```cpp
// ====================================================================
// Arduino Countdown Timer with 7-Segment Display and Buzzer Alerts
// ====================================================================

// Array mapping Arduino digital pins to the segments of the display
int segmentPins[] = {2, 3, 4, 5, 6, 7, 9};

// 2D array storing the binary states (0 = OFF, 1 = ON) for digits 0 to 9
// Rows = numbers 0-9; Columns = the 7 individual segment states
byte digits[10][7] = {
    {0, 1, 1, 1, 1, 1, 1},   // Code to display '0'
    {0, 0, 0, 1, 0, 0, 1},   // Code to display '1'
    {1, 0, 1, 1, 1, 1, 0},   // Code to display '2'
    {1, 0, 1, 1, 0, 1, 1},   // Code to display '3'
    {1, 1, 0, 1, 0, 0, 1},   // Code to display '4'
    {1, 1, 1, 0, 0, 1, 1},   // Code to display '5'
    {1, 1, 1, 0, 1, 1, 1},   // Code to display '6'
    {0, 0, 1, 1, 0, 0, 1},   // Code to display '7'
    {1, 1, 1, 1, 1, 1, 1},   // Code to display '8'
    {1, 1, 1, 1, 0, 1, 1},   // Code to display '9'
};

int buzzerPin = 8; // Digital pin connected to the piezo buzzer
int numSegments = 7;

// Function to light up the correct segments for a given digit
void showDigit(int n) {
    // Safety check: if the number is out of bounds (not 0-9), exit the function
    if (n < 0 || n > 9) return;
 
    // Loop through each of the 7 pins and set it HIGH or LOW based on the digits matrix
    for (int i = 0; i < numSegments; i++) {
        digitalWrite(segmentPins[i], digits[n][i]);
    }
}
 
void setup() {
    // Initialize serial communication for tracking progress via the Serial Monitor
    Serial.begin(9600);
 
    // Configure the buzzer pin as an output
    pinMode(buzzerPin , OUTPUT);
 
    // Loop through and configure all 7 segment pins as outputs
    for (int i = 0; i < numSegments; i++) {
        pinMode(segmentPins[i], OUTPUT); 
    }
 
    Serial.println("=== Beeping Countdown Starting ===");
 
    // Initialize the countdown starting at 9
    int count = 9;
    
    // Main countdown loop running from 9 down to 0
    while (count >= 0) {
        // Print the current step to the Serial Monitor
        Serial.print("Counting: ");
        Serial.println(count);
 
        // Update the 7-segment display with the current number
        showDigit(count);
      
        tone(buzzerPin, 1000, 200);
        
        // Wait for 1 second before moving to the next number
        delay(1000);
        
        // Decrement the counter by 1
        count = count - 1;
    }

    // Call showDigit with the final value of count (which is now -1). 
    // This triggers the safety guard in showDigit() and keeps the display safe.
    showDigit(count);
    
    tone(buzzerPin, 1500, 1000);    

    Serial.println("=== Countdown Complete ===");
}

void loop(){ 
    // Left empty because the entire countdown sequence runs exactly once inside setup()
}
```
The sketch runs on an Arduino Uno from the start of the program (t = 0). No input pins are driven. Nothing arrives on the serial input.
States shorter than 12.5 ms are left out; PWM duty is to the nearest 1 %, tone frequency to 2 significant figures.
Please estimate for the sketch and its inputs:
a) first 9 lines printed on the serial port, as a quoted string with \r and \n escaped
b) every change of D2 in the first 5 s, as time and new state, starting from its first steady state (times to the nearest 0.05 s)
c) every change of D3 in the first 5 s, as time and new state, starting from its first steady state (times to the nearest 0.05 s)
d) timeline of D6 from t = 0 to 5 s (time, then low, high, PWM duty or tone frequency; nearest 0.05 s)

"=== Beeping Countdown Starting ===\r\nCounting: 9\r\nCounting: 8\r\nCounting: 7\r\nCounting: 6\r\nCounting: 5\r\nCounting: 4\r\nCounting: 3\r\nCounting: 2\r\n"
0 s high; 2 s low; 3 s high
0 s high; 2 s low; 3 s high
0 s low; 1 s high; 2 s low; 3 s high; 4 s low
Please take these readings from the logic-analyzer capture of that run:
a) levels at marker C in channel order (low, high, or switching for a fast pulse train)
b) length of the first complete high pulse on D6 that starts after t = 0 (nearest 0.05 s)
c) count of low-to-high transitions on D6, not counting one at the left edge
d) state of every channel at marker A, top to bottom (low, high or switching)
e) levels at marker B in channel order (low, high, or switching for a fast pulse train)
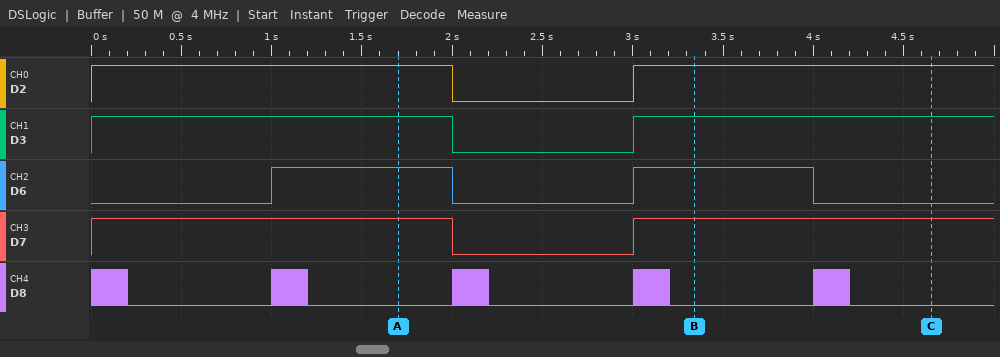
D2 high, D3 high, D6 low, D7 high, D8 low
1.00 s
2
D2 high, D3 high, D6 high, D7 high, D8 low
D2 high, D3 high, D6 high, D7 high, D8 low
